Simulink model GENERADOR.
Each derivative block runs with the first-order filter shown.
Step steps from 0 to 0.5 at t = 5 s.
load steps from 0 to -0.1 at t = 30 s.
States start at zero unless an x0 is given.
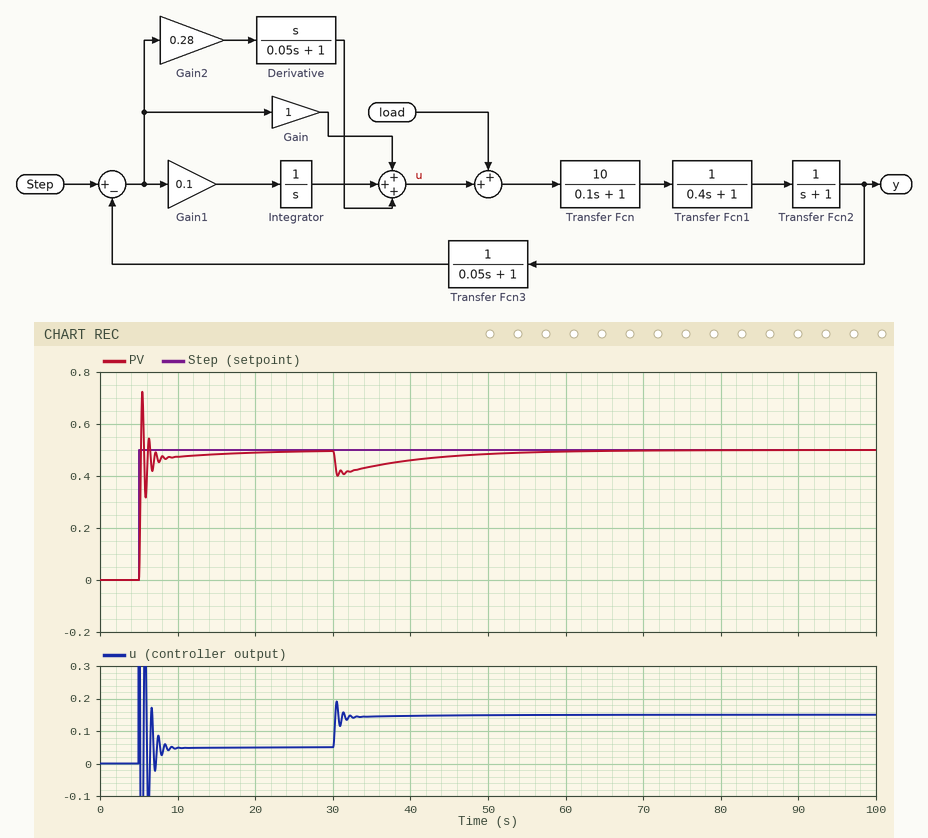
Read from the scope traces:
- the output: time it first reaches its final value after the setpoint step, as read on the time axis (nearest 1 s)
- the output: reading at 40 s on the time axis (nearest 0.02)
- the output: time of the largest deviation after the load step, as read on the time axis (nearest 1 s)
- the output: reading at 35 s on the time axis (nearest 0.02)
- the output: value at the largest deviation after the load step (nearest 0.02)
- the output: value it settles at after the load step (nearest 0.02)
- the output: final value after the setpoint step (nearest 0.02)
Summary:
5 s
0.46
31 s
0.44
0.40
0.50
0.50
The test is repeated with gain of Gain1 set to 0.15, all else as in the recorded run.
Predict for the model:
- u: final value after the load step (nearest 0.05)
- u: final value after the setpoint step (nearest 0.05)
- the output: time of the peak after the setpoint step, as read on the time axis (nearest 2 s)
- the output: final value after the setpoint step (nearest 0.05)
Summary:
0.15
0.05
6 s
0.50
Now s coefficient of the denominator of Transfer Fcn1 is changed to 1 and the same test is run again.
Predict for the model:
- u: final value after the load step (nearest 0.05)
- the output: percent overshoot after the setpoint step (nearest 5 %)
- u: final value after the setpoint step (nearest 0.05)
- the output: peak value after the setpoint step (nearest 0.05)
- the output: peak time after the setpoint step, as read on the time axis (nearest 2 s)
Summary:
0.15
25 %
0.05
0.65
6 s
